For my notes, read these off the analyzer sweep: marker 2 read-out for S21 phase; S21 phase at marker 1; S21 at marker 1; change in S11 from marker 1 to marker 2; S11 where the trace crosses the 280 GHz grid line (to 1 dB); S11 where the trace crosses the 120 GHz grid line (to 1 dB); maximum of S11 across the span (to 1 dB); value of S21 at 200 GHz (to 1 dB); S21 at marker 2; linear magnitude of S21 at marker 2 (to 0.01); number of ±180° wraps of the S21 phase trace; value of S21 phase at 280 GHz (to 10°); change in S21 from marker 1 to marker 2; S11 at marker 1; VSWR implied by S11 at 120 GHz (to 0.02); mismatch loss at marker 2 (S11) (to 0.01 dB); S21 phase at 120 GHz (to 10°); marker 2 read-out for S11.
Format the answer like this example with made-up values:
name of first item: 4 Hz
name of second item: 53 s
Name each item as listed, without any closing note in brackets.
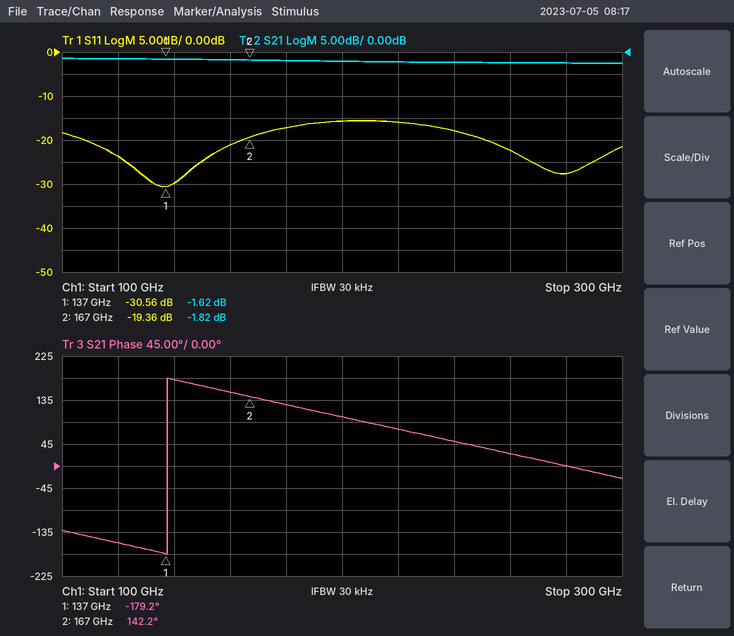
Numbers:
marker 2 read-out for S21 phase: 142.2°
S21 phase at marker 1: -179.2°
S21 at marker 1: -1.62 dB
change in S11 from marker 1 to marker 2: 11.20 dB
S11 where the trace crosses the 280 GHz grid line: -28 dB
S11 where the trace crosses the 120 GHz grid line: -24 dB
maximum of S11 across the span: -16 dB
value of S21 at 200 GHz: -2 dB
S21 at marker 2: -1.82 dB
linear magnitude of S21 at marker 2: 0.81
number of ±180° wraps of the S21 phase trace: 1
value of S21 phase at 280 GHz: 0°
change in S21 from marker 1 to marker 2: -0.20 dB
S11 at marker 1: -30.56 dB
VSWR implied by S11 at 120 GHz: 1.14
mismatch loss at marker 2 (S11): 0.05 dB
S21 phase at 120 GHz: -160°
marker 2 read-out for S11: -19.36 dB
